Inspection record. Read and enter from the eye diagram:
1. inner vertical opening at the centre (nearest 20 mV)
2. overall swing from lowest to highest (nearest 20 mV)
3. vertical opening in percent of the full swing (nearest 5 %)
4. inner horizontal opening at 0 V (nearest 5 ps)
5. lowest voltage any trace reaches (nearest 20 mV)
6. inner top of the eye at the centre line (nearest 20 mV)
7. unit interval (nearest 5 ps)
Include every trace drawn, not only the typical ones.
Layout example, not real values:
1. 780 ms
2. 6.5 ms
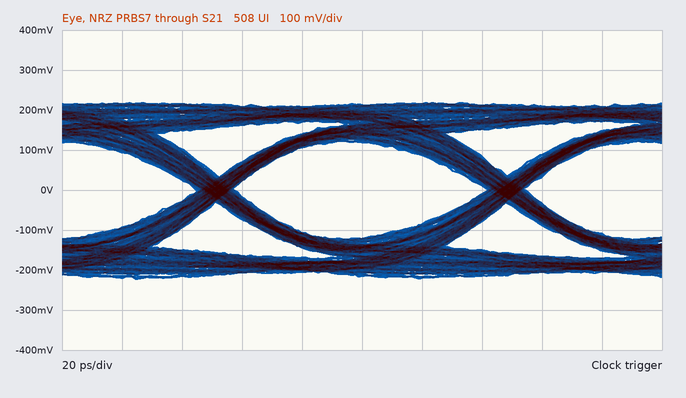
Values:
1. 240 mV
2. 440 mV
3. 55 %
4. 85 ps
5. -220 mV
6. 120 mV
7. 95 ps
